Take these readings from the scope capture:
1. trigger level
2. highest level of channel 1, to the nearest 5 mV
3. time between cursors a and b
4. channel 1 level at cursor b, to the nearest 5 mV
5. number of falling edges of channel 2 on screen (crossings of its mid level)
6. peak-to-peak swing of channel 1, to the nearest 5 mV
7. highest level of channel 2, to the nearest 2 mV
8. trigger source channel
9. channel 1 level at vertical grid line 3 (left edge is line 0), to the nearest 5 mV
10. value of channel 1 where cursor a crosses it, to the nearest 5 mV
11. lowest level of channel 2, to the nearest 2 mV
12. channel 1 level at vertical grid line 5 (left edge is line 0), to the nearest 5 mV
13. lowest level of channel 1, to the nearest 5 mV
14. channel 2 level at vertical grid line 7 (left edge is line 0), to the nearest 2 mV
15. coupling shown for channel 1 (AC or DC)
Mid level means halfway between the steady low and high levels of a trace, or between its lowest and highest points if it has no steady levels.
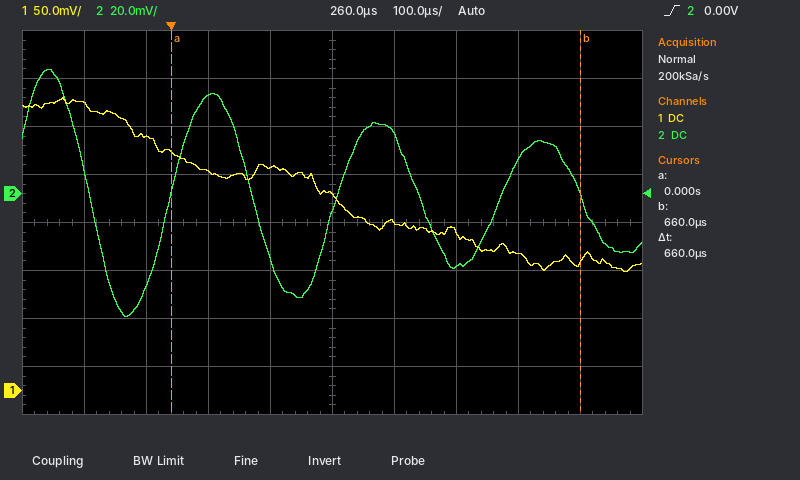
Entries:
0.00 V
305 mV
660 µs
135 mV
4
180 mV
52 mV
channel 2
230 mV
250 mV
-52 mV
205 mV
125 mV
-30 mV
DC
